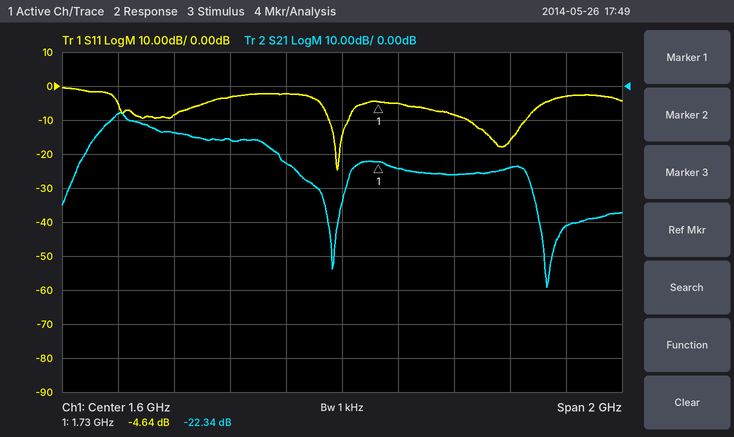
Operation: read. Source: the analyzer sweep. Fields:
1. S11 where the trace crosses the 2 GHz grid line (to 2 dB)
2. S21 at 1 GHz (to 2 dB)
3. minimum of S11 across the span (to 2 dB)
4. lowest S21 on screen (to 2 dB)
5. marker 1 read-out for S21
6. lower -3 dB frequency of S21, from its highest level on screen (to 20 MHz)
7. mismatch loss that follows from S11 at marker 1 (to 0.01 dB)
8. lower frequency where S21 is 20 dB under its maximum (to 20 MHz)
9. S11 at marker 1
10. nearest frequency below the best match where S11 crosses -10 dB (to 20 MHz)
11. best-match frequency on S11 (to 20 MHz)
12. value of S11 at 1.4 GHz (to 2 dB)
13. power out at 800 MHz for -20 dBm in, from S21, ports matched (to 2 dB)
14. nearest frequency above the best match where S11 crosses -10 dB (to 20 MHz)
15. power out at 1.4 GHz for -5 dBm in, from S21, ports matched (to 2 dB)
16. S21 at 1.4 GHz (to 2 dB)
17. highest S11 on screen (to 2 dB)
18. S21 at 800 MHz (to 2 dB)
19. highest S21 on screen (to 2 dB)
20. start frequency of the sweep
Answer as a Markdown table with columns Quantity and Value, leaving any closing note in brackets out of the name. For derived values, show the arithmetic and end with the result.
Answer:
| Quantity | Value |
|---|---|
| S11 where the trace crosses the 2 GHz grid line | -8 dB |
| S21 at 1 GHz | -14 dB |
| minimum of S11 across the span | -24 dB |
| lowest S21 on screen | -60 dB |
| marker 1 read-out for S21 | -22.34 dB |
| lower -3 dB frequency of S21, from its highest level on screen | 760 MHz |
| mismatch loss that follows from S11 at marker 1 | −10 log10(1 − 10^(-4.64/10)) ≈ 1.83 dB |
| lower frequency where S21 is 20 dB under its maximum | 640 MHz |
| S11 at marker 1 | -4.64 dB |
| nearest frequency below the best match where S11 crosses -10 dB | 1.56 GHz |
| best-match frequency on S11 | 1.58 GHz |
| value of S11 at 1.4 GHz | -2 dB |
| power out at 800 MHz for -20 dBm in, from S21, ports matched | -20 dBm + (-8 dB) = -28 dBm |
| nearest frequency above the best match where S11 crosses -10 dB | 1.62 GHz |
| power out at 1.4 GHz for -5 dBm in, from S21, ports matched | -5 dBm + (-22 dB) = -28 dBm |
| S21 at 1.4 GHz | -22 dB |
| highest S11 on screen | 0 dB |
| S21 at 800 MHz | -8 dB |
| highest S21 on screen | -8 dB |
| start frequency of the sweep | 600 MHz |
